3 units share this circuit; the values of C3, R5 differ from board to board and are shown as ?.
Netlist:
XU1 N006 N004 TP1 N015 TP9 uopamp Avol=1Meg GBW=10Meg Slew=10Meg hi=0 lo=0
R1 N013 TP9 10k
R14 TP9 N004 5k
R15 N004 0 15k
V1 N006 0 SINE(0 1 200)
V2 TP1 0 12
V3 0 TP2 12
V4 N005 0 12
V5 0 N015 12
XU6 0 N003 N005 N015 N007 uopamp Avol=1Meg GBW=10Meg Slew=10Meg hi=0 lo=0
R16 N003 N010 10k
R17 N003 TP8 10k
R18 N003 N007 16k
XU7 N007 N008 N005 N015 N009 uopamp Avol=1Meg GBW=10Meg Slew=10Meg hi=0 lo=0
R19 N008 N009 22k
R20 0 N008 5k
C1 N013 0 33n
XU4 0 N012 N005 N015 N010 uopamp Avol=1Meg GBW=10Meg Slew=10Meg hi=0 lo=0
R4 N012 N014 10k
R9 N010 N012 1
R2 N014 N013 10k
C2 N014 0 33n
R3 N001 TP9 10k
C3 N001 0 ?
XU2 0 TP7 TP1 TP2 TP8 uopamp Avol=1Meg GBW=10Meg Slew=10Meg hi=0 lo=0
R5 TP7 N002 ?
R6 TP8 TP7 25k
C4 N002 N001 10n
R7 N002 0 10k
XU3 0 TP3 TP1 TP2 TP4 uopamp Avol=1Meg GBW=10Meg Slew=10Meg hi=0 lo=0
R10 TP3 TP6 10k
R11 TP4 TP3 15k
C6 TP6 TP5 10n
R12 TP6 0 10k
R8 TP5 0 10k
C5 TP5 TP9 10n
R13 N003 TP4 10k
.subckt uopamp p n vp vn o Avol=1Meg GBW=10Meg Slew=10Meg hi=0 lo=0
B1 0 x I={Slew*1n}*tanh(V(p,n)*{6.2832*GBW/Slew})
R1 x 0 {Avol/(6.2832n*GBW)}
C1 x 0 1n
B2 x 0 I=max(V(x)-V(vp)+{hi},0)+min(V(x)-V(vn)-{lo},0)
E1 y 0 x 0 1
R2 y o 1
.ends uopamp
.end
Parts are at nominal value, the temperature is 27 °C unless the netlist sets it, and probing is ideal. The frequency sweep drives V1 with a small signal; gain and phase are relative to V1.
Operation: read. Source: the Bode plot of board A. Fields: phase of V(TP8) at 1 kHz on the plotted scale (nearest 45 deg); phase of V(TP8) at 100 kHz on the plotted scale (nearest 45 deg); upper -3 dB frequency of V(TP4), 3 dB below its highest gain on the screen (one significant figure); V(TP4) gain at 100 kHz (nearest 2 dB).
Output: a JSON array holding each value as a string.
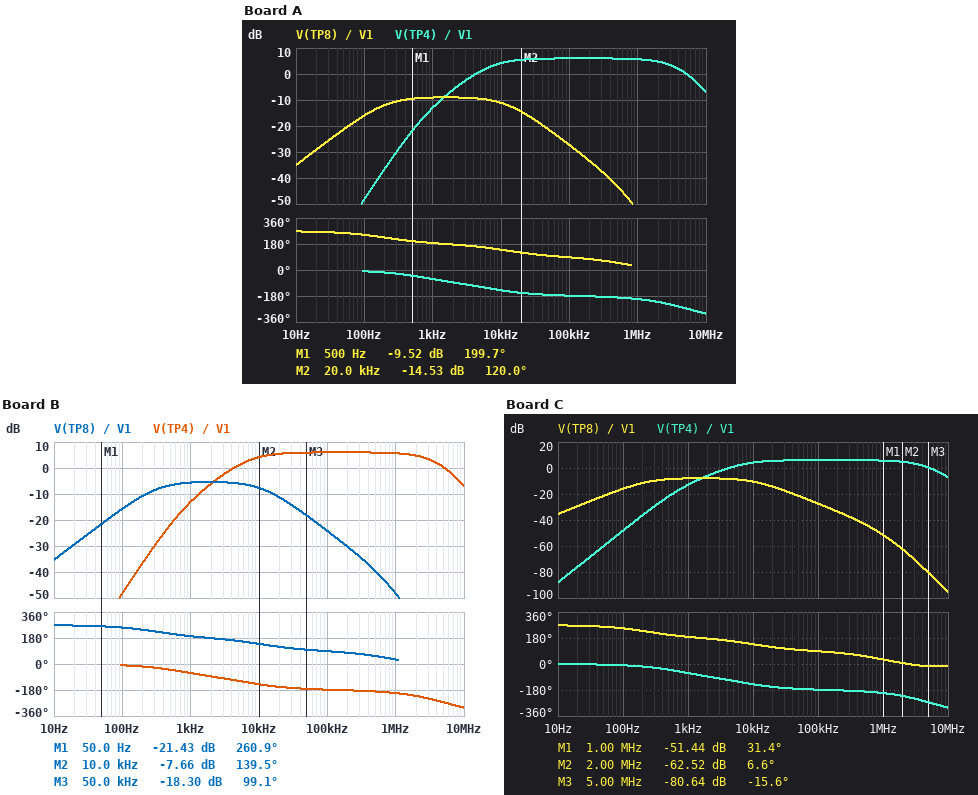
["180 deg", "90 deg", "3 MHz", "6 dB"]
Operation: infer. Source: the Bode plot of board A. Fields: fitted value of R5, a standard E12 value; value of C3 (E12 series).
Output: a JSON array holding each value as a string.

["1.8 kΩ", "68 nF"]
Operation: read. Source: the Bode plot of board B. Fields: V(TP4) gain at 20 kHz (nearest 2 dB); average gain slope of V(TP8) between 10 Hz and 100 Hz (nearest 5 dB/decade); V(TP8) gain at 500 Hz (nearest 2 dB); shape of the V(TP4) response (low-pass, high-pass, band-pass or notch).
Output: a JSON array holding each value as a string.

["6 dB", "20 dB/decade", "-6 dB", "band-pass"]
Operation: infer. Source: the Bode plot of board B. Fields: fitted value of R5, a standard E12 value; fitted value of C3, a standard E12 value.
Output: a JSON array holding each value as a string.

["2.2 kΩ", "39 nF"]
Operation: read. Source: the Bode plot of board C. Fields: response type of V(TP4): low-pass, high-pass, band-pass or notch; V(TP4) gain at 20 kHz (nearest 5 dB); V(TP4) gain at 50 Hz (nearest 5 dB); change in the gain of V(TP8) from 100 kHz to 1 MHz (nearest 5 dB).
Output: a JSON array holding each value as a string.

["band-pass", "5 dB", "-60 dB", "-25 dB"]
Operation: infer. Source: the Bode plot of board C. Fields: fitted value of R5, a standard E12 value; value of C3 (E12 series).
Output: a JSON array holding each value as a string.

["2.2 kΩ", "56 nF"]
